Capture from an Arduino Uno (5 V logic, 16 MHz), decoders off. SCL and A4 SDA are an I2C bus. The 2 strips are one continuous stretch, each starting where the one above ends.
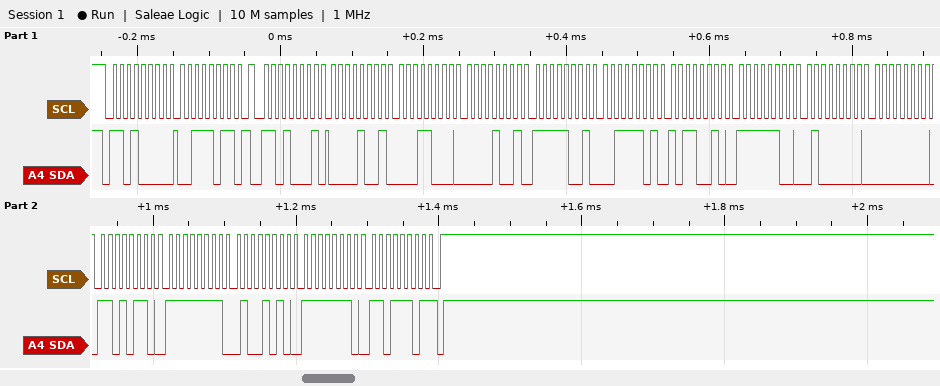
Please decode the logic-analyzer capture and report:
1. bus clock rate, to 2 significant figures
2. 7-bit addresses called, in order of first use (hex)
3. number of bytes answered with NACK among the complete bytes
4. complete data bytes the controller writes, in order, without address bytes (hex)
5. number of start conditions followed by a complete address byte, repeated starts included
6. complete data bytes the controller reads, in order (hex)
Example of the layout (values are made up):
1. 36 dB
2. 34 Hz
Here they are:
1. 100 kHz
2. 0x68
3. 1
4. 3B
5. 2
6. 09 18 09 F9 3D B2 FC 40 00 D6 FF 4A FE DD
